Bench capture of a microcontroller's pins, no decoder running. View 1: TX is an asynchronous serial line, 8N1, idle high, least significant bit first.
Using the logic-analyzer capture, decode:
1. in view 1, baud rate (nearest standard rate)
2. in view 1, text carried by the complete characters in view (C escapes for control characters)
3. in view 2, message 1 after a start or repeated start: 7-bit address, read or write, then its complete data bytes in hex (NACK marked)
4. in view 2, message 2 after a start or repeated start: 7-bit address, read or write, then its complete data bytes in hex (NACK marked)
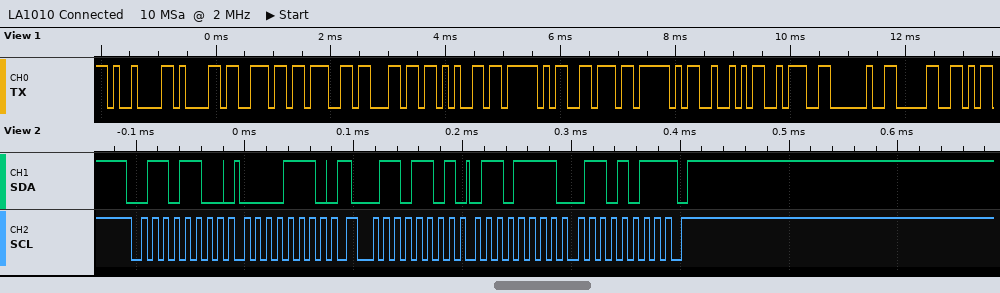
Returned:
9600 baud
"\tangle_v_R: 0"
0x36 write: 0E
0x36 read: 6F 6B NACK
